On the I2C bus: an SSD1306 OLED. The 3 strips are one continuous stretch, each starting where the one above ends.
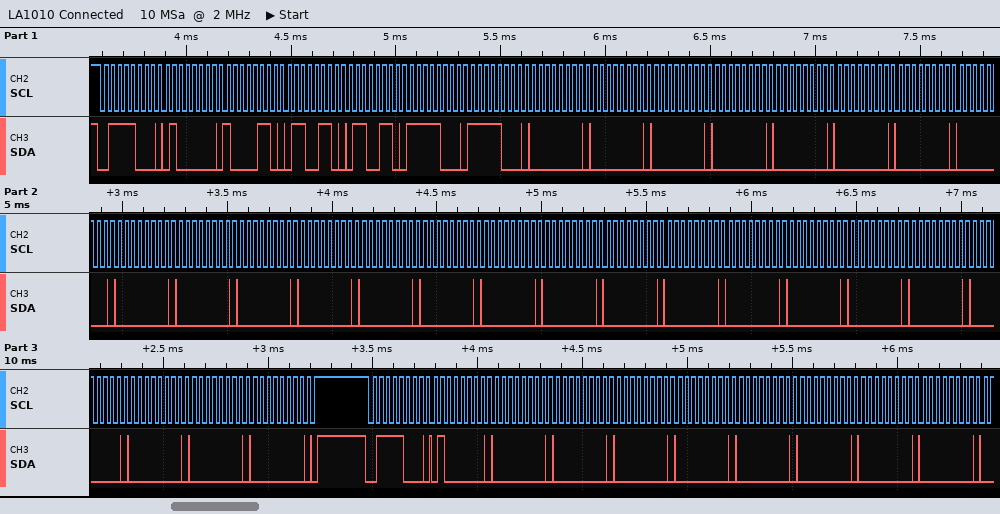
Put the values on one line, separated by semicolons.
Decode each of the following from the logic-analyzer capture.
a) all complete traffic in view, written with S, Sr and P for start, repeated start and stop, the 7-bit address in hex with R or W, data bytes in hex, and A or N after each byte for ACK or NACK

S 3CW A 40 A 86 A 66 A 66 A F8 A F8 A 00 A 00 A 00 A 00 A 00 A 00 A 00 A 00 A 00 A 00 A 00 A 00 A 00 A 00 A 00 A 00 A 00 A 00 A 00 A 00 A 00 A 00 A 00 A 00 A 00 A 00 A P S 3CW A 40 A 00 A 00 A 00 A 00 A 00 A 00 A 00 A 00 A
